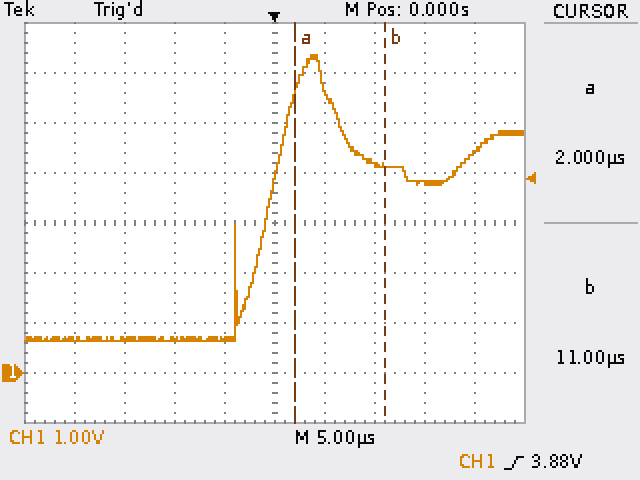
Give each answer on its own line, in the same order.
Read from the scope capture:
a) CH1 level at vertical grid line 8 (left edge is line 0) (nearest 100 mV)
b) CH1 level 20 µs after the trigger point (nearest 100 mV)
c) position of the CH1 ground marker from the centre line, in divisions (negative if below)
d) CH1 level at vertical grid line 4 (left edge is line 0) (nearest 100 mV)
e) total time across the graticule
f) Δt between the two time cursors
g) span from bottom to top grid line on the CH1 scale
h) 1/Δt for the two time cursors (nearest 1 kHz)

3.8 V
4.4 V
-3.0 div
700 mV
50 µs
9.0 µs
8 V
111 kHz
